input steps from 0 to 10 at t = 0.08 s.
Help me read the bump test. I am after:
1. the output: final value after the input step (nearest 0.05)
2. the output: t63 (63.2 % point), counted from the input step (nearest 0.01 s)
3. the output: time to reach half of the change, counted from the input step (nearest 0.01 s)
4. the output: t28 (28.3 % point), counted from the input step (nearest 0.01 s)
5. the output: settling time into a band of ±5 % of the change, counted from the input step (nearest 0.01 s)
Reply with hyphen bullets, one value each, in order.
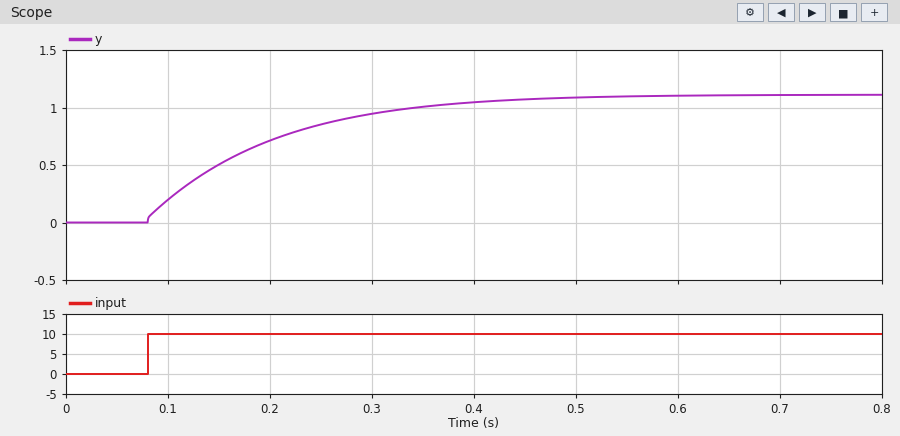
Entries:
- 1.10
- 0.12 s
- 0.08 s
- 0.04 s
- 0.34 s
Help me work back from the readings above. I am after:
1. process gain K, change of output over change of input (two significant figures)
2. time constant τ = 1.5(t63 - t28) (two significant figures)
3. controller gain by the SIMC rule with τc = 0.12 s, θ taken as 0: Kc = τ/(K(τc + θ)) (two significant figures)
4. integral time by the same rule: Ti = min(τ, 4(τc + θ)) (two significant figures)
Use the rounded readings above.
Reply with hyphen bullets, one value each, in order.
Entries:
- 0.11
- 0.12 s
- 9.1
- 0.12 s
